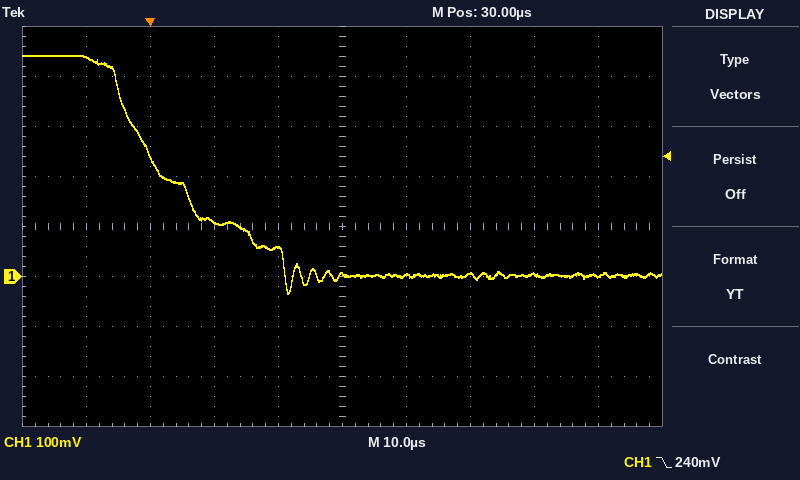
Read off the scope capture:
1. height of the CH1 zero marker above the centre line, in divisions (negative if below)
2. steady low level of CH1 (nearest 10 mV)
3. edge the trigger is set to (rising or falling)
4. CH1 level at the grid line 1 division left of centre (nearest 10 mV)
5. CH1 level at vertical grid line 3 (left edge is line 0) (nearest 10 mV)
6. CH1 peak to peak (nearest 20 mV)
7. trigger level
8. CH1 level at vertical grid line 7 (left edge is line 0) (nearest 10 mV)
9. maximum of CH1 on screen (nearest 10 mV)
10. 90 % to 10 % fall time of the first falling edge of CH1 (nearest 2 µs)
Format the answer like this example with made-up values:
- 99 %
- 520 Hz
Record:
- -1.0 div
- 0 mV
- falling
- 60 mV
- 110 mV
- 480 mV
- 240 mV
- 10 mV
- 440 mV
- 26 µs
